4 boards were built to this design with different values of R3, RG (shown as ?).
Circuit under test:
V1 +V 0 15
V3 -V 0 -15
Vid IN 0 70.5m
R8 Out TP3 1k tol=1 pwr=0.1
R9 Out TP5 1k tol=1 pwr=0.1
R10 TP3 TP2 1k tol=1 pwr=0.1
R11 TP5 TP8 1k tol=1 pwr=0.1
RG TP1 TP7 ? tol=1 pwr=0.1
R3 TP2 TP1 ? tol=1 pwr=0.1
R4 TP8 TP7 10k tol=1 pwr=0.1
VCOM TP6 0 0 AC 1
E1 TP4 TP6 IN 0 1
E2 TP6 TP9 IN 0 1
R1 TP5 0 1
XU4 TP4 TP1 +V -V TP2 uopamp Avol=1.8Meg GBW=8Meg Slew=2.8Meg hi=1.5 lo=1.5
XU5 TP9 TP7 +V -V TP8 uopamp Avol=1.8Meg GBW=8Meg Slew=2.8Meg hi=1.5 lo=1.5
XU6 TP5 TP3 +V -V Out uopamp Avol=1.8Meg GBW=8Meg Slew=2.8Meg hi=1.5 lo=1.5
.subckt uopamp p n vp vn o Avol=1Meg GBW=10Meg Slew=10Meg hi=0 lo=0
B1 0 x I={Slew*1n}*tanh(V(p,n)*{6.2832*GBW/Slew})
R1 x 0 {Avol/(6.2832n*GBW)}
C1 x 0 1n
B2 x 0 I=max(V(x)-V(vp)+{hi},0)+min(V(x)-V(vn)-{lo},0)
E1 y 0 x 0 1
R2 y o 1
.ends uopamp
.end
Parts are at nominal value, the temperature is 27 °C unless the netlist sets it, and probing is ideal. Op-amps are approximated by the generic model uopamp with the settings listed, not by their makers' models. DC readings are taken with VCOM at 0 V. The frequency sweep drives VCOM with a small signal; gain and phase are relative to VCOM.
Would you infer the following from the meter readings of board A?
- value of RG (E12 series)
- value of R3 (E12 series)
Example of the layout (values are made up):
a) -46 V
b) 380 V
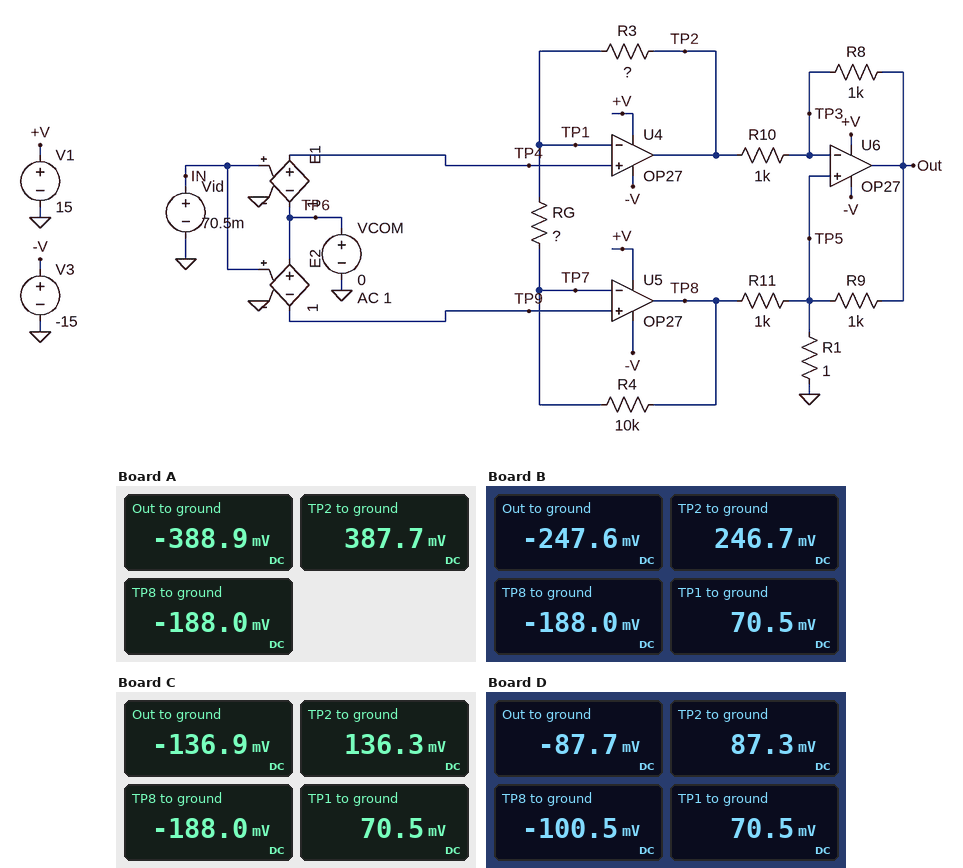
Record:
a) 12 kΩ
b) 27 kΩ
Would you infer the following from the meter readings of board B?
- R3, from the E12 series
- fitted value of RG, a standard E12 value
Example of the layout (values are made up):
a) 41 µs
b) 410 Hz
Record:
a) 15 kΩ
b) 12 kΩ
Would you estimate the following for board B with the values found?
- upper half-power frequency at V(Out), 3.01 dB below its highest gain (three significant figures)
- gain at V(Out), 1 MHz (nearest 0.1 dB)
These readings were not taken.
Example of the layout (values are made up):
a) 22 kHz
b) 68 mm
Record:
a) 3.34 MHz
b) -0.3 dB
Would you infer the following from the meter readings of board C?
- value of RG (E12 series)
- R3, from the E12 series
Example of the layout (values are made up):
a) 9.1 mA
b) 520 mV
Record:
a) 12 kΩ
b) 5.6 kΩ
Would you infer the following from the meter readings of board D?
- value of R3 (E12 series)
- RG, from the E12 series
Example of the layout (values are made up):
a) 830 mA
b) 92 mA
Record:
a) 5.6 kΩ
b) 47 kΩ
